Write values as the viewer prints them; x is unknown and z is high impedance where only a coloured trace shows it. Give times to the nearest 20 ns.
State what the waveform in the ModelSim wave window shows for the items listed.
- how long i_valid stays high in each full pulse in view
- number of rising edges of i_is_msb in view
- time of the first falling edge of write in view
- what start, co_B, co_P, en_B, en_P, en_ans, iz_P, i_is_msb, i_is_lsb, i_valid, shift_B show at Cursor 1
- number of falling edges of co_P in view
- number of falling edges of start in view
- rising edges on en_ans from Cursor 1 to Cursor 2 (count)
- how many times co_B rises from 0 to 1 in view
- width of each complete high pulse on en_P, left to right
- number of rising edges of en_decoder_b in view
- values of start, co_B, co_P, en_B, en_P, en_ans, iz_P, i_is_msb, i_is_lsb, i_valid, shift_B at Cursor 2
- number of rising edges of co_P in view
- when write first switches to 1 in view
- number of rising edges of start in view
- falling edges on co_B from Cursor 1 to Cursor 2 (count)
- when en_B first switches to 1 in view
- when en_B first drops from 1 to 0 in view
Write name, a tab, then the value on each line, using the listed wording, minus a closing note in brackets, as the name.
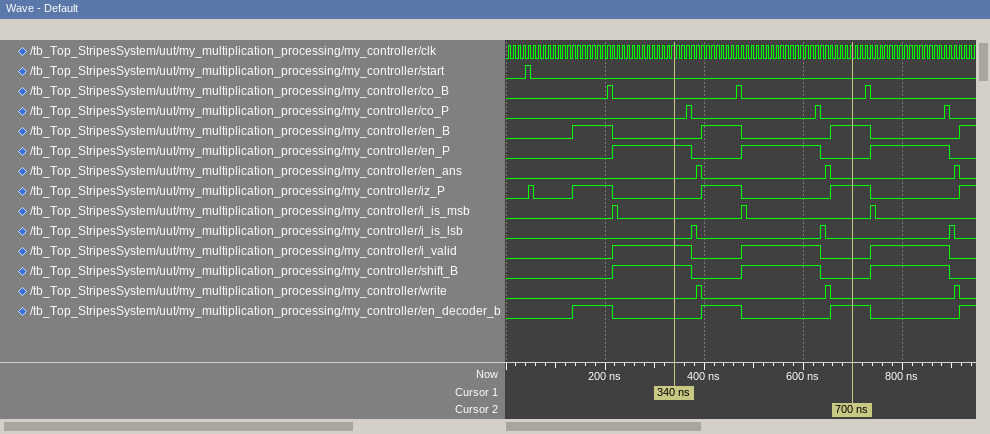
how long i_valid stays high in each full pulse in view	160 ns, 160 ns, 160 ns
number of rising edges of i_is_msb in view	3
time of the first falling edge of write in view	400 ns
what start, co_B, co_P, en_B, en_P, en_ans, iz_P, i_is_msb, i_is_lsb, i_valid, shift_B show at Cursor 1	start=0, co_B=0, co_P=0, en_B=0, en_P=1, en_ans=0, iz_P=0, i_is_msb=0, i_is_lsb=0, i_valid=1, shift_B=1
number of falling edges of co_P in view	3
number of falling edges of start in view	1
rising edges on en_ans from Cursor 1 to Cursor 2	2
how many times co_B rises from 0 to 1 in view	3
width of each complete high pulse on en_P, left to right	160 ns, 160 ns, 160 ns
number of rising edges of en_decoder_b in view	4
values of start, co_B, co_P, en_B, en_P, en_ans, iz_P, i_is_msb, i_is_lsb, i_valid, shift_B at Cursor 2	start=0, co_B=0, co_P=0, en_B=1, en_P=0, en_ans=0, iz_P=1, i_is_msb=0, i_is_lsb=0, i_valid=0, shift_B=0
number of rising edges of co_P in view	3
when write first switches to 1 in view	380 ns
number of rising edges of start in view	1
falling edges on co_B from Cursor 1 to Cursor 2	1
when en_B first switches to 1 in view	140 ns
when en_B first drops from 1 to 0 in view	220 ns
